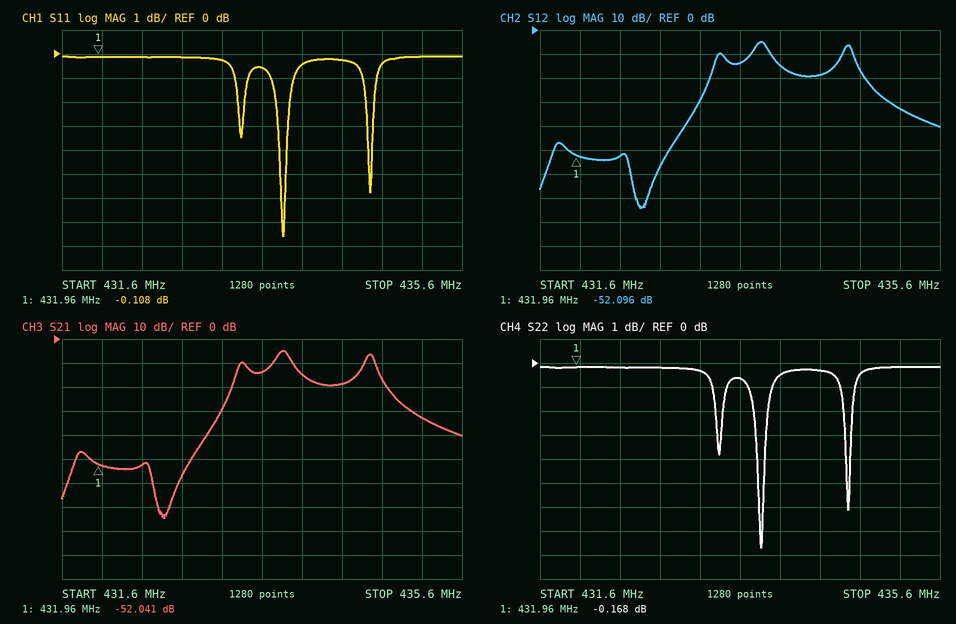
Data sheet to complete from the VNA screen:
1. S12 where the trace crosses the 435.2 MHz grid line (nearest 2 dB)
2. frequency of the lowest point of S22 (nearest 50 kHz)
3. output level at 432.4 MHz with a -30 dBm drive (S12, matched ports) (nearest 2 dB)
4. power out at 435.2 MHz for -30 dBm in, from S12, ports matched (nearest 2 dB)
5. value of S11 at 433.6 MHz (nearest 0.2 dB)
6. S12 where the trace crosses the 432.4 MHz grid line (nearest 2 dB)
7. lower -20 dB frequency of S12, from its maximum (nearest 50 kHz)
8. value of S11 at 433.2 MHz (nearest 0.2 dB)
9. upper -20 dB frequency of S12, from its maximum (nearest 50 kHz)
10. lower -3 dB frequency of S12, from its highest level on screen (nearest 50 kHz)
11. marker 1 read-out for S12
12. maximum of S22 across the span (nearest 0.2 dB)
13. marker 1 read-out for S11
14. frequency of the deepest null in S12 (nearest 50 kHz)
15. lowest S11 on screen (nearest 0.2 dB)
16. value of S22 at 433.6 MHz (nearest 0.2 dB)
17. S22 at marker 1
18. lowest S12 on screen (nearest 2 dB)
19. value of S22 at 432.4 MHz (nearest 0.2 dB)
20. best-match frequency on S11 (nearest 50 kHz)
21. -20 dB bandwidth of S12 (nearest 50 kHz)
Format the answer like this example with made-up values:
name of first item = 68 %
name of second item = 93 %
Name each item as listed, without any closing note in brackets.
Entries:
S12 where the trace crosses the 435.2 MHz grid line = -32 dB
frequency of the lowest point of S22 = 433.80 MHz
output level at 432.4 MHz with a -30 dBm drive (S12, matched ports) = -82 dBm
power out at 435.2 MHz for -30 dBm in, from S12, ports matched = -62 dBm
value of S11 at 433.6 MHz = -0.6 dB
S12 where the trace crosses the 432.4 MHz grid line = -52 dB
lower -20 dB frequency of S12, from its maximum = 433.25 MHz
value of S11 at 433.2 MHz = -0.2 dB
upper -20 dB frequency of S12, from its maximum = 434.95 MHz
lower -3 dB frequency of S12, from its highest level on screen = 433.75 MHz
marker 1 read-out for S12 = -52.096 dB
maximum of S22 across the span = -0.2 dB
marker 1 read-out for S11 = -0.108 dB
frequency of the deepest null in S12 = 432.60 MHz
lowest S11 on screen = -7.6 dB
value of S22 at 433.6 MHz = -0.6 dB
S22 at marker 1 = -0.168 dB
lowest S12 on screen = -74 dB
value of S22 at 432.4 MHz = -0.2 dB
best-match frequency on S11 = 433.80 MHz
-20 dB bandwidth of S12 = 1.70 MHz
